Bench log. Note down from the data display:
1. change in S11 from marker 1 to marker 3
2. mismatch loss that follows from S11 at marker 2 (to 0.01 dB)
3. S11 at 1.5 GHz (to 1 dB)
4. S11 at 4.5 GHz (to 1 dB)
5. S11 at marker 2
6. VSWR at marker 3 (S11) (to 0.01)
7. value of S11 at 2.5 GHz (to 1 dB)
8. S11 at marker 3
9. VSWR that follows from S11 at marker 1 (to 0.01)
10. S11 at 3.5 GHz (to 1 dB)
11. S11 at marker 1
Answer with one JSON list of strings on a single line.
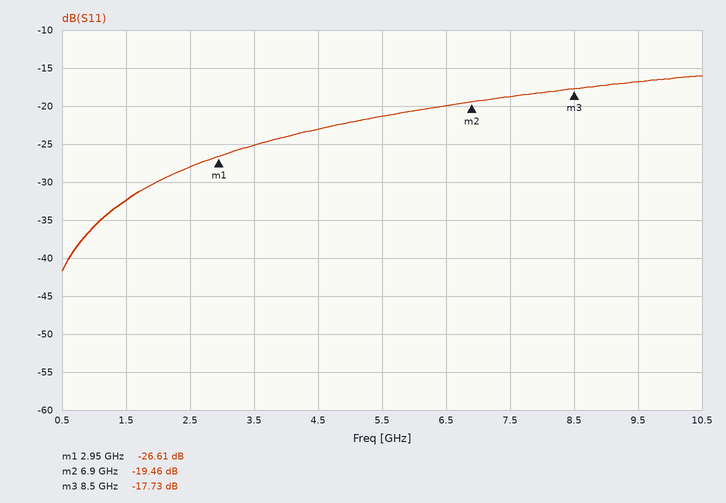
["8.88 dB", "0.05 dB", "-32 dB", "-23 dB", "-19.46 dB", "1.30", "-28 dB", "-17.73 dB", "1.10", "-25 dB", "-26.61 dB"]
